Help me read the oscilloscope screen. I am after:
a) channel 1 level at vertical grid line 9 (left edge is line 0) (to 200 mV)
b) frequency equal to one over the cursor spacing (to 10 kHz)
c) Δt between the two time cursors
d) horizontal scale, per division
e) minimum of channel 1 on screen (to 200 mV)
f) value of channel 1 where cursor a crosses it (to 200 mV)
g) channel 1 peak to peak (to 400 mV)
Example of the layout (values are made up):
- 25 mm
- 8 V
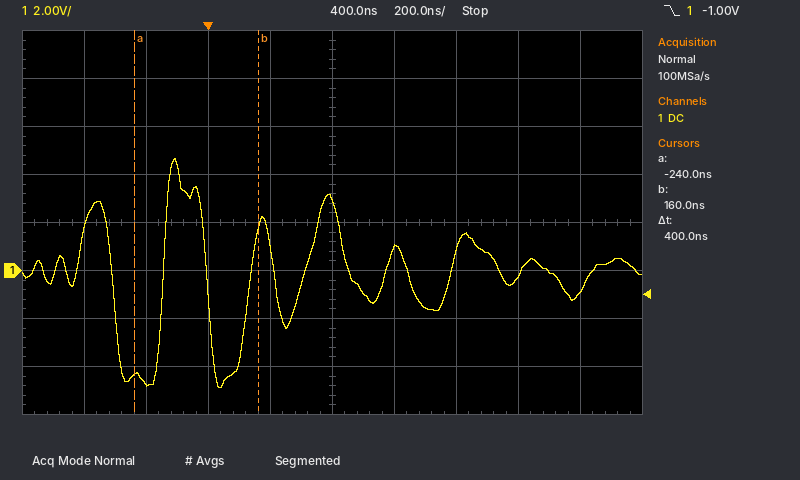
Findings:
- -800 mV
- 2.50 MHz
- 400 ns
- 200 ns
- -4.8 V
- -4.4 V
- 9.6 V
